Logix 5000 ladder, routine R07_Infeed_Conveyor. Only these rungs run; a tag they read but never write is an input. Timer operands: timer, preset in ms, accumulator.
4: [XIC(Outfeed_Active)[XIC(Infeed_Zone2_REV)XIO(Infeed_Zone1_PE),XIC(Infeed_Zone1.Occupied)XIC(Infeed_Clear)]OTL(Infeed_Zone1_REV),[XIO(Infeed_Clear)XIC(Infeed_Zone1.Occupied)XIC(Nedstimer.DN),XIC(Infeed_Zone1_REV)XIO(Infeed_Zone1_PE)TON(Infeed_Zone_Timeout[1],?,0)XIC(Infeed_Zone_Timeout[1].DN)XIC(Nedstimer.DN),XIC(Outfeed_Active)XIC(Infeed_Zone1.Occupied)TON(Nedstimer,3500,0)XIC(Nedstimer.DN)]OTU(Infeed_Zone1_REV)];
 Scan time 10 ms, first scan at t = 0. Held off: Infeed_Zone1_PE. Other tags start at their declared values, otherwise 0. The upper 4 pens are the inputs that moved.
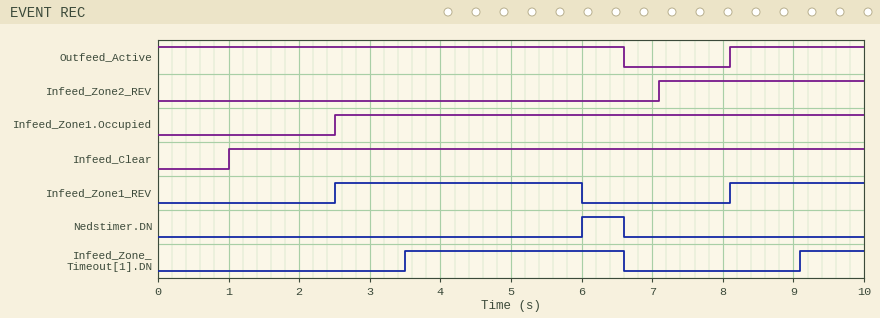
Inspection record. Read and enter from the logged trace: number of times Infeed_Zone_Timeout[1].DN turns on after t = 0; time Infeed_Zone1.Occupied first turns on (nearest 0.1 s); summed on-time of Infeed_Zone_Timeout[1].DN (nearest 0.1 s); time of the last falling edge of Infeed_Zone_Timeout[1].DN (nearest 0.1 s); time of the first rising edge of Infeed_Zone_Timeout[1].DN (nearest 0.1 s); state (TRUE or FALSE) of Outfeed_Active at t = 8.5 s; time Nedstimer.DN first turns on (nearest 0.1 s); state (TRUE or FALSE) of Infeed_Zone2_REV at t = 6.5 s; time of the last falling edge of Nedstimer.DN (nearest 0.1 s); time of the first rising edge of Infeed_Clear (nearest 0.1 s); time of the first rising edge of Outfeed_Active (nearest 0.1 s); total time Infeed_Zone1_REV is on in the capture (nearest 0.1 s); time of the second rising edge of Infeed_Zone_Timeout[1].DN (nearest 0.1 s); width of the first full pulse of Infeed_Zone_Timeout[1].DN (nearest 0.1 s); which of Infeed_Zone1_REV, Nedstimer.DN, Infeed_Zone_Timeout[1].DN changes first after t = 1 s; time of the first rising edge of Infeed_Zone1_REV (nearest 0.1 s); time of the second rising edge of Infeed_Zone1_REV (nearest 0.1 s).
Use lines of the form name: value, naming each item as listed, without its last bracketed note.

number of times Infeed_Zone_Timeout[1].DN turns on after t = 0: 2
time Infeed_Zone1.Occupied first turns on: 2.5 s
summed on-time of Infeed_Zone_Timeout[1].DN: 4.0 s
time of the last falling edge of Infeed_Zone_Timeout[1].DN: 6.6 s
time of the first rising edge of Infeed_Zone_Timeout[1].DN: 3.5 s
state (TRUE or FALSE) of Outfeed_Active at t = 8.5 s: TRUE
time Nedstimer.DN first turns on: 6.0 s
state (TRUE or FALSE) of Infeed_Zone2_REV at t = 6.5 s: FALSE
time of the last falling edge of Nedstimer.DN: 6.6 s
time of the first rising edge of Infeed_Clear: 1.0 s
time of the first rising edge of Outfeed_Active: 8.1 s
total time Infeed_Zone1_REV is on in the capture: 5.4 s
time of the second rising edge of Infeed_Zone_Timeout[1].DN: 9.1 s
width of the first full pulse of Infeed_Zone_Timeout[1].DN: 3.1 s
which of Infeed_Zone1_REV, Nedstimer.DN, Infeed_Zone_Timeout[1].DN changes first after t = 1 s: Infeed_Zone1_REV
time of the first rising edge of Infeed_Zone1_REV: 2.5 s
time of the second rising edge of Infeed_Zone1_REV: 8.1 s
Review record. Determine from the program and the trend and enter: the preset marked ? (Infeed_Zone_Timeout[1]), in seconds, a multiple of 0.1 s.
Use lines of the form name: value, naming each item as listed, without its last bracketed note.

the preset marked ? (Infeed_Zone_Timeout[1]), in seconds, a multiple of 0.1 s: 1.0 s
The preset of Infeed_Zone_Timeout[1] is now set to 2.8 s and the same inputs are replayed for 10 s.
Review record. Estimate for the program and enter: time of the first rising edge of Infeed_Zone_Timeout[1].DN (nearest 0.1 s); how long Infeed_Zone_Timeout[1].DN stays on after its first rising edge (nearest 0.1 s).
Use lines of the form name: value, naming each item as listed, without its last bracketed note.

time of the first rising edge of Infeed_Zone_Timeout[1].DN: 5.3 s
how long Infeed_Zone_Timeout[1].DN stays on after its first rising edge: 1.3 s
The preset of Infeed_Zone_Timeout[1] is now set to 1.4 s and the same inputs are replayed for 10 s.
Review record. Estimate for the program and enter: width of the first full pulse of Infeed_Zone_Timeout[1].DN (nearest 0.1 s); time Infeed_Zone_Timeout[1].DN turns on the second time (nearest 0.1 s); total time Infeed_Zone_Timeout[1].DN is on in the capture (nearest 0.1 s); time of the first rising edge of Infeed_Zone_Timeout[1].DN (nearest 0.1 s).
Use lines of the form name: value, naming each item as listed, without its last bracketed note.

width of the first full pulse of Infeed_Zone_Timeout[1].DN: 2.7 s
time Infeed_Zone_Timeout[1].DN turns on the second time: 9.5 s
total time Infeed_Zone_Timeout[1].DN is on in the capture: 3.2 s
time of the first rising edge of Infeed_Zone_Timeout[1].DN: 3.9 s
